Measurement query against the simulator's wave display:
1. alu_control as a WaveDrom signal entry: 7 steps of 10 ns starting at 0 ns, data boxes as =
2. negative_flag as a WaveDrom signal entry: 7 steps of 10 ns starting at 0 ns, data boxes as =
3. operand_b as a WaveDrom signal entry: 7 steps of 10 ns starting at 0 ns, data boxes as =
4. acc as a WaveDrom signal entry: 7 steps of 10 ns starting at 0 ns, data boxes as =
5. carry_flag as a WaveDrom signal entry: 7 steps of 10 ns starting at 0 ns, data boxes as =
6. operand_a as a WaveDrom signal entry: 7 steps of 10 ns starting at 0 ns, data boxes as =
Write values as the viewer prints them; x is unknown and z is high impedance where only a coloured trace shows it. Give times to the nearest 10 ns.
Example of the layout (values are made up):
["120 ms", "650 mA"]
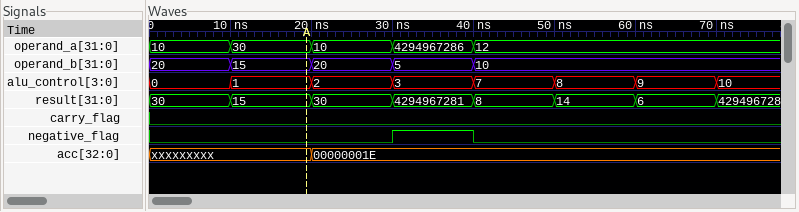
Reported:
["{name: 'alu_control', wave: '=======', data: '0 1 2 3 7 8 9'}", "{name: 'negative_flag', wave: '0..10..'}", "{name: 'operand_b', wave: '=====..', data: '20 15 20 5 10'}", "{name: 'acc', wave: 'x.=....', data: '00000001E'}", "{name: 'carry_flag', wave: '0......'}", "{name: 'operand_a', wave: '=====..', data: '10 30 10 4294967286 12'}"]
